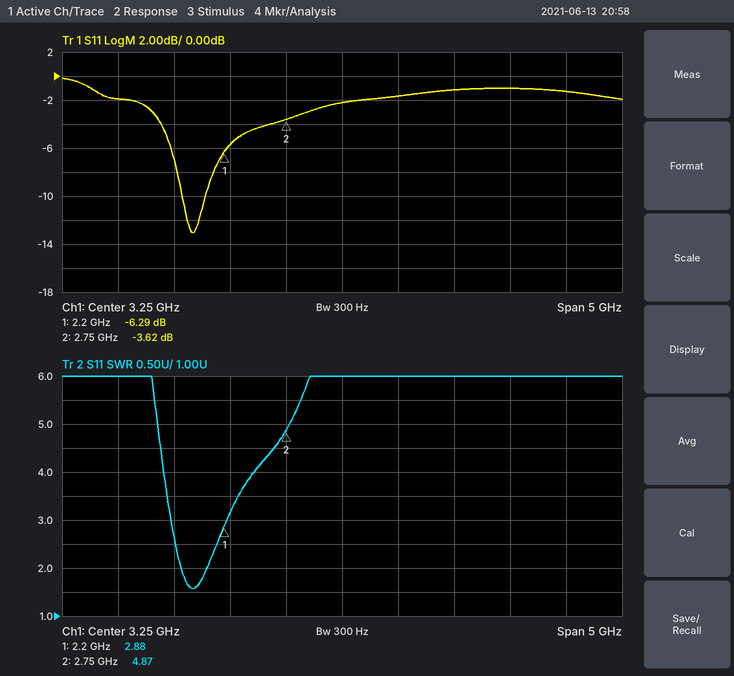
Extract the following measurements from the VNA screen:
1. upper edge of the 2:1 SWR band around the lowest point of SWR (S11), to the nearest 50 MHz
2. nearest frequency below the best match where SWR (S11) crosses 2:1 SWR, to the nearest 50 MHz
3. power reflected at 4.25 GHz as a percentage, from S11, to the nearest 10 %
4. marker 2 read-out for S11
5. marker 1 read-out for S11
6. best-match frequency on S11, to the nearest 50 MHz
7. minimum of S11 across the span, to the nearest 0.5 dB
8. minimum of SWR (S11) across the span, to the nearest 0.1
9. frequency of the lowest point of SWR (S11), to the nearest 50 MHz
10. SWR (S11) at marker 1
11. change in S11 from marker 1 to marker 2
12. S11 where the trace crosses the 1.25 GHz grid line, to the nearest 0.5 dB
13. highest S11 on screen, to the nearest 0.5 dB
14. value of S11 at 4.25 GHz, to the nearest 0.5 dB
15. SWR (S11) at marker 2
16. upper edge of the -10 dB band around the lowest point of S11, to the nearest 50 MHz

2.05 GHz
1.80 GHz
80 %
-3.62 dB
-6.29 dB
1.90 GHz
-13.0 dB
1.6
1.90 GHz
2.88
2.67 dB
-2.0 dB
0.0 dB
-1.0 dB
4.87
2.05 GHz
